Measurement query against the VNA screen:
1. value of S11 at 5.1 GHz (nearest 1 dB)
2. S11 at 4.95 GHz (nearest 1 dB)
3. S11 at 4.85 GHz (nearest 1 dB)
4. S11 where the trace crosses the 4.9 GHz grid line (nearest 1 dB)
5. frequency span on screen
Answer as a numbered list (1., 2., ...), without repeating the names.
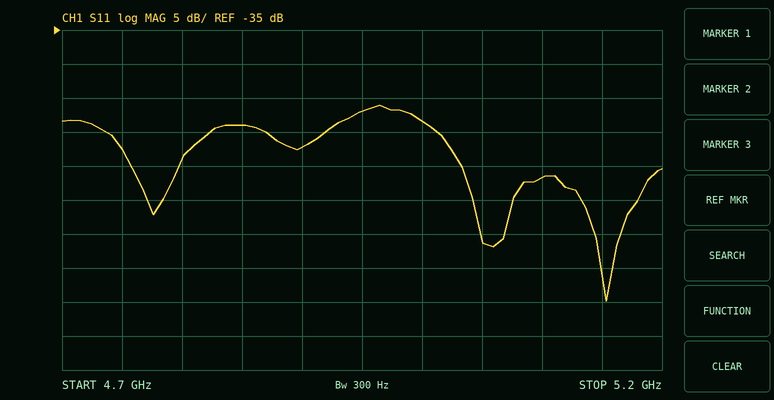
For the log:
1. -57 dB
2. -47 dB
3. -49 dB
4. -52 dB
5. 500 MHz
